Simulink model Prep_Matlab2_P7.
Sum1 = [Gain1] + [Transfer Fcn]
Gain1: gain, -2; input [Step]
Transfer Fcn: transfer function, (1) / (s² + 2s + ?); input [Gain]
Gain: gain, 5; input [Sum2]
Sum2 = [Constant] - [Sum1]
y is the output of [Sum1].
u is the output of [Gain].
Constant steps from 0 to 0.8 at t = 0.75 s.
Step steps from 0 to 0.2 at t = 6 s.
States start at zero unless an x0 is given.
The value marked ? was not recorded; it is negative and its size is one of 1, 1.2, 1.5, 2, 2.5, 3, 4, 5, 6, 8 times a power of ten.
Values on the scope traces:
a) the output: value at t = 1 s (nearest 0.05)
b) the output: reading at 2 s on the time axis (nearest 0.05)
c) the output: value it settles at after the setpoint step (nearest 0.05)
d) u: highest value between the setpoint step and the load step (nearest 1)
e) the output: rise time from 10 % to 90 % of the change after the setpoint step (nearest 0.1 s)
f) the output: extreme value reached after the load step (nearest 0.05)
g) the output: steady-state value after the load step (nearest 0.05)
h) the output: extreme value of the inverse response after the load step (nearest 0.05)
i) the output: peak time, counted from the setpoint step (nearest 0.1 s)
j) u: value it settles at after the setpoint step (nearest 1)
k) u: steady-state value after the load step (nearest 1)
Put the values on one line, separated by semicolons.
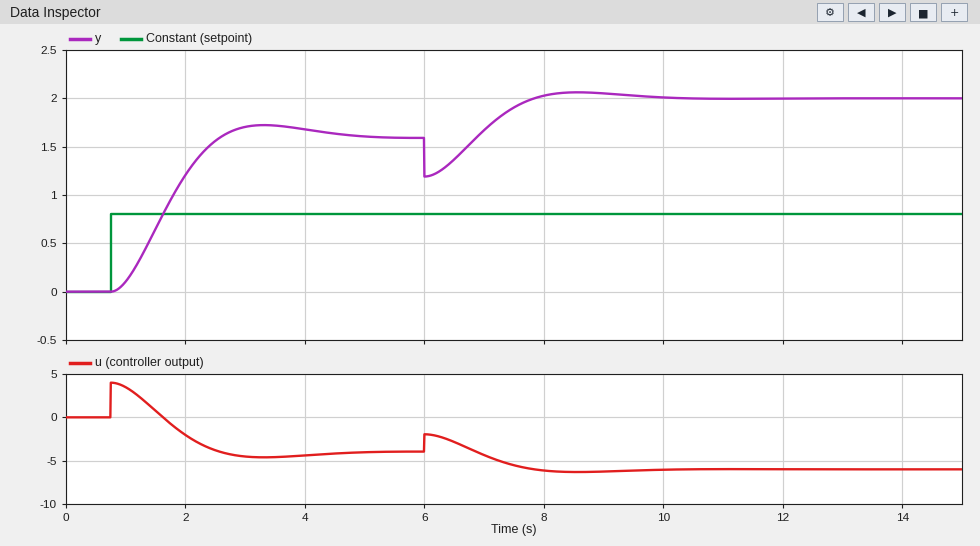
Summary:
0.10; 1.20; 1.60; 4; 1.2 s; 2.05; 2.00; 1.20; 2.6 s; -4; -6
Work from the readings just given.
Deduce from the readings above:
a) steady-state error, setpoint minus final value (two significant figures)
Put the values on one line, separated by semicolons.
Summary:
-0.80
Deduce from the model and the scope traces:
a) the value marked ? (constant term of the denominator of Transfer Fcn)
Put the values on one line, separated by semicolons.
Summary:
-2.5
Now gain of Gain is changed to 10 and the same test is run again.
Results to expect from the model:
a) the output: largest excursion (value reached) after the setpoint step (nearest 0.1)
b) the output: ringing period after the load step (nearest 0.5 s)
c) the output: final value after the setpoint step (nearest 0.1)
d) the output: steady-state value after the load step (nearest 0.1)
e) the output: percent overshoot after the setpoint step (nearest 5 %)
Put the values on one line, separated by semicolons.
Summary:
1.4; 2.5 s; 1.1; 1.2; 30 %
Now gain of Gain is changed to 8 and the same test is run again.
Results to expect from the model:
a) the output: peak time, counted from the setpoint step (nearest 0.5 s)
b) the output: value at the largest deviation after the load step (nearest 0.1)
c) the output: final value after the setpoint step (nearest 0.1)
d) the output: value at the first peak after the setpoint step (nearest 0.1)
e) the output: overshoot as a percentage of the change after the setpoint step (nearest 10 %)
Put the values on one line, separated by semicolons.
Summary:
1.5 s; 1.5; 1.2; 1.4; 20 %
